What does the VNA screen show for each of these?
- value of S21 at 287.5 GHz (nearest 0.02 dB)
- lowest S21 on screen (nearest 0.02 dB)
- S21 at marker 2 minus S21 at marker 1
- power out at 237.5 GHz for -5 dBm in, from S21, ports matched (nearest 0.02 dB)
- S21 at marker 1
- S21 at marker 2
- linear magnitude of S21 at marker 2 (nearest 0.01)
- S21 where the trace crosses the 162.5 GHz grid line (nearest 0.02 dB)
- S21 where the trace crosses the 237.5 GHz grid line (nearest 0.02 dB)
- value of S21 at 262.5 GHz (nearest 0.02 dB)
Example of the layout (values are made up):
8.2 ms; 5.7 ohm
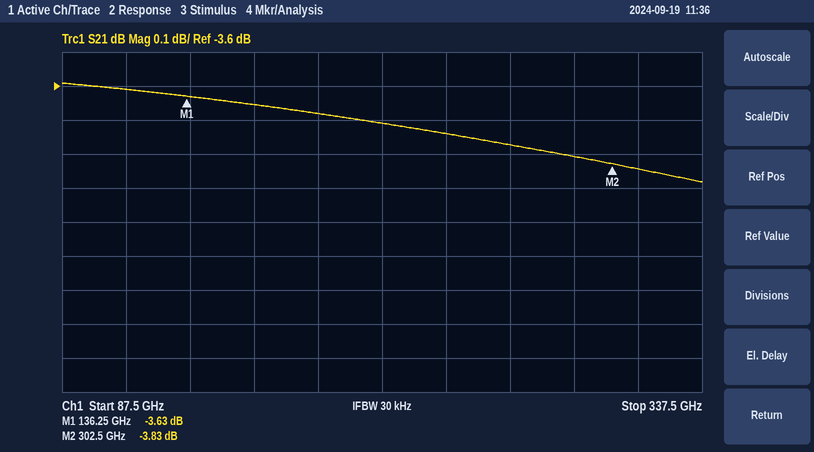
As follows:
-3.80 dB; -3.88 dB; -0.20 dB; -8.74 dBm; -3.63 dB; -3.83 dB; 0.64; -3.66 dB; -3.74 dB; -3.78 dB
